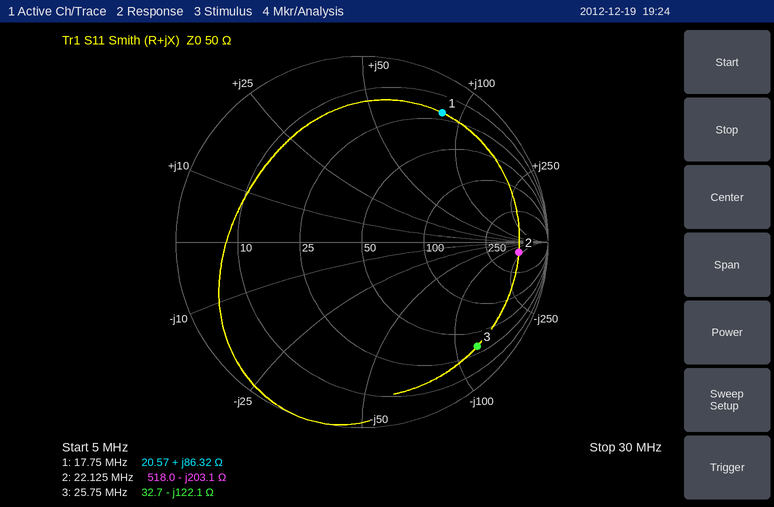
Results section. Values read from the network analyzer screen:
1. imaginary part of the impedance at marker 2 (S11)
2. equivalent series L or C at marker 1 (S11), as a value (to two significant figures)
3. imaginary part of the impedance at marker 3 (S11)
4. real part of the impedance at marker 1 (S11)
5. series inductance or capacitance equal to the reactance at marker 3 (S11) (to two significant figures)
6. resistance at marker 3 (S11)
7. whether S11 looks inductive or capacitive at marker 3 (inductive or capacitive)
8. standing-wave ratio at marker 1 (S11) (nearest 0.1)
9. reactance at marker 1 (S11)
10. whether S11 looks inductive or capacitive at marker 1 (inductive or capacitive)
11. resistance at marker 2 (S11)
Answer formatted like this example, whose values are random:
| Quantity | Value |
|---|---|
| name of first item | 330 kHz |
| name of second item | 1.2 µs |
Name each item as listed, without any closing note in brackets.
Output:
| Quantity | Value |
|---|---|
| imaginary part of the impedance at marker 2 | -203.1 Ω |
| equivalent series L or C at marker 1 (S11), as a value | 770 nH |
| imaginary part of the impedance at marker 3 | -122.1 Ω |
| real part of the impedance at marker 1 | 20.57 Ω |
| series inductance or capacitance equal to the reactance at marker 3 (S11) | 51 pF |
| resistance at marker 3 | 32.7 Ω |
| whether S11 looks inductive or capacitive at marker 3 | capacitive |
| standing-wave ratio at marker 1 (S11) | 10.0 |
| reactance at marker 1 | +86.32 Ω |
| whether S11 looks inductive or capacitive at marker 1 | inductive |
| resistance at marker 2 | 518.0 Ω |
